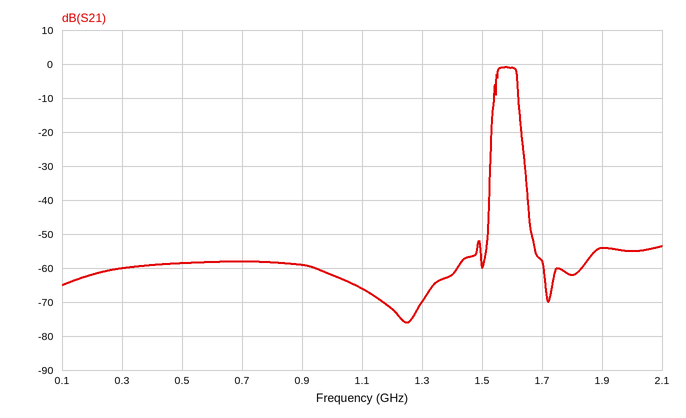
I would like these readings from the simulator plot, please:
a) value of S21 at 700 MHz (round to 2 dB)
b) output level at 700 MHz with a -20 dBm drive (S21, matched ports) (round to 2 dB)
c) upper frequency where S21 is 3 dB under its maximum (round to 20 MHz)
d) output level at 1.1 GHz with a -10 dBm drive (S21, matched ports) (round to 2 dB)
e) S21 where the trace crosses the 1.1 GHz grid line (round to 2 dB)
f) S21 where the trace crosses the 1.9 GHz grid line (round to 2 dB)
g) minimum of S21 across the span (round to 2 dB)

-58 dB
-78 dBm
1.62 GHz
-76 dBm
-66 dB
-54 dB
-76 dB
